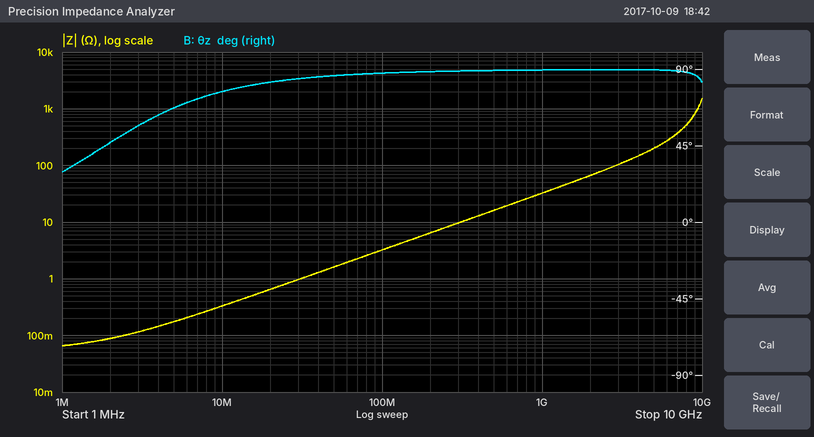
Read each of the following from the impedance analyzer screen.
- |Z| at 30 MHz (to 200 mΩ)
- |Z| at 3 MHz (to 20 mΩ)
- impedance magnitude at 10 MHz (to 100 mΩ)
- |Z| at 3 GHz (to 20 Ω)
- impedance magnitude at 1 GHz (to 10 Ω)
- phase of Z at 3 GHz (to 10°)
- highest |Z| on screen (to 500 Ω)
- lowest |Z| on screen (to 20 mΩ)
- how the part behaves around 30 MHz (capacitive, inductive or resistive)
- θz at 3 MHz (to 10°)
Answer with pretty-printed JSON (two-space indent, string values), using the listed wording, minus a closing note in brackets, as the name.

{
  "|Z| at 30 MHz": "1.0 Ω",
  "|Z| at 3 MHz": "120 mΩ",
  "impedance magnitude at 10 MHz": "300 mΩ",
  "|Z| at 3 GHz": "100 Ω",
  "impedance magnitude at 1 GHz": "30 Ω",
  "phase of Z at 3 GHz": "90°",
  "highest |Z| on screen": "1.5 kΩ",
  "lowest |Z| on screen": "60 mΩ",
  "how the part behaves around 30 MHz": "inductive",
  "θz at 3 MHz": "60°"
}
